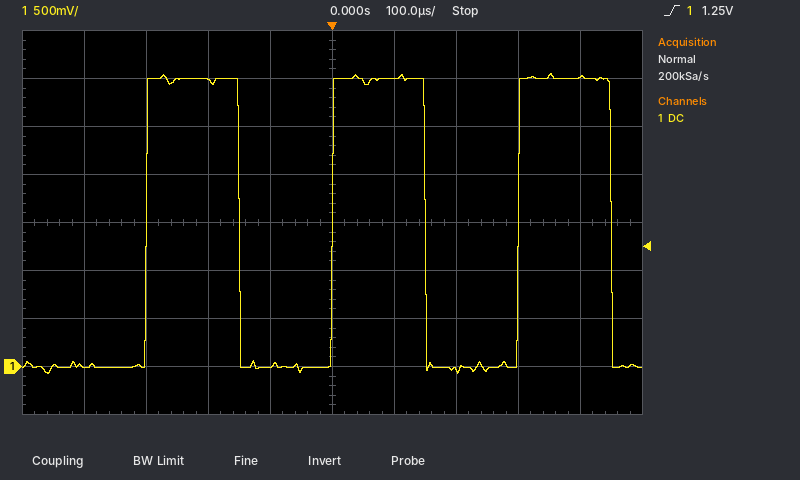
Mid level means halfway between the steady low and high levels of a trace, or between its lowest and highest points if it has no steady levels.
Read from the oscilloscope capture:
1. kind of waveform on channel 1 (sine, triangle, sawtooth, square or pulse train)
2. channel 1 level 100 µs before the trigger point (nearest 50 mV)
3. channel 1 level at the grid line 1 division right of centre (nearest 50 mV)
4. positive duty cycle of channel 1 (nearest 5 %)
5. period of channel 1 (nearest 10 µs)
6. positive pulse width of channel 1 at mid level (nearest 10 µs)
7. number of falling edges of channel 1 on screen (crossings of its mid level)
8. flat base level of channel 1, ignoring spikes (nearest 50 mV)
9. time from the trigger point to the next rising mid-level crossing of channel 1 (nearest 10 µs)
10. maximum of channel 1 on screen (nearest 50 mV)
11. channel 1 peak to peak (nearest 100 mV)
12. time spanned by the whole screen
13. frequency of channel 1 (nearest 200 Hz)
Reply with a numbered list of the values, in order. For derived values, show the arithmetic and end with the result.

1. square
2. 0 mV
3. 3.00 V
4. 150 µs / 300 µs ≈ 50 %
5. 300 µs
6. 150 µs
7. 3
8. 0 mV
9. 300 µs
10. 3.05 V
11. 3.10 V
12. 1 ms
13. 1 / 300 µs ≈ 3.33 kHz, so 3.4 kHz to the nearest 200 Hz
